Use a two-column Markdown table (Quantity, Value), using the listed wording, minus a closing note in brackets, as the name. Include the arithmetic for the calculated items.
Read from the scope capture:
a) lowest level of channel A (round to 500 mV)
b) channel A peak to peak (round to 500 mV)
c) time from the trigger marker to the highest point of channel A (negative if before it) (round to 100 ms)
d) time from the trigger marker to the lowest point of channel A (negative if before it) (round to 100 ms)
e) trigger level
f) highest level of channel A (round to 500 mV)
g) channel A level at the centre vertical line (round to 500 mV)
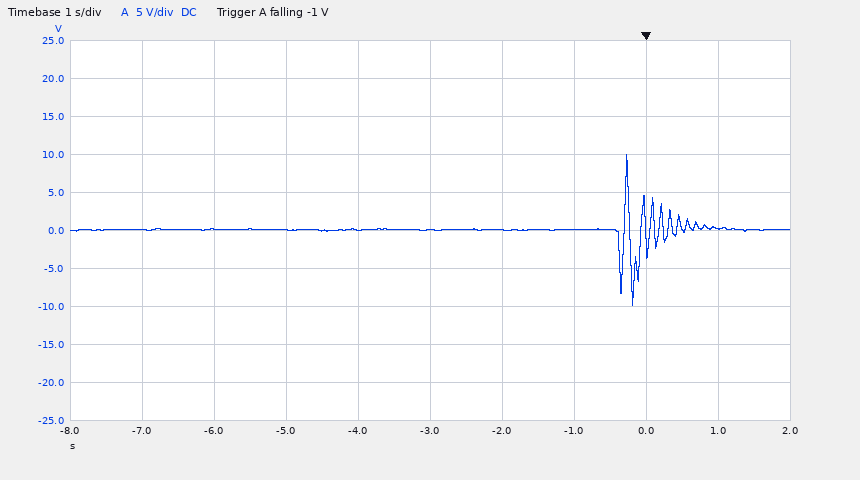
| Quantity | Value |
|---|---|
| lowest level of channel A | -10.0 V |
| channel A peak to peak | 10.0 V − (-10.0 V) = 20.0 V |
| time from the trigger marker to the highest point of channel A (negative if before it) | -300 ms |
| time from the trigger marker to the lowest point of channel A (negative if before it) | -200 ms |
| trigger level | -1 V |
| highest level of channel A | 10.0 V |
| channel A level at the centre vertical line | 0.0 V |
